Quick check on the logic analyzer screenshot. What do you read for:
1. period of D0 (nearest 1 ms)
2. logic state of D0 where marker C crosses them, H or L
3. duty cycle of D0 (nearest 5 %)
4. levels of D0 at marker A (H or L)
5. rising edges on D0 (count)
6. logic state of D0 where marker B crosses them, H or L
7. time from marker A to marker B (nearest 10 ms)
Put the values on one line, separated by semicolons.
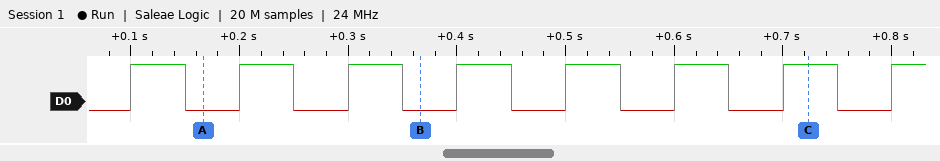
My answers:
100 ms; D0=H; 50 %; D0=L; 8; D0=L; 200 ms
